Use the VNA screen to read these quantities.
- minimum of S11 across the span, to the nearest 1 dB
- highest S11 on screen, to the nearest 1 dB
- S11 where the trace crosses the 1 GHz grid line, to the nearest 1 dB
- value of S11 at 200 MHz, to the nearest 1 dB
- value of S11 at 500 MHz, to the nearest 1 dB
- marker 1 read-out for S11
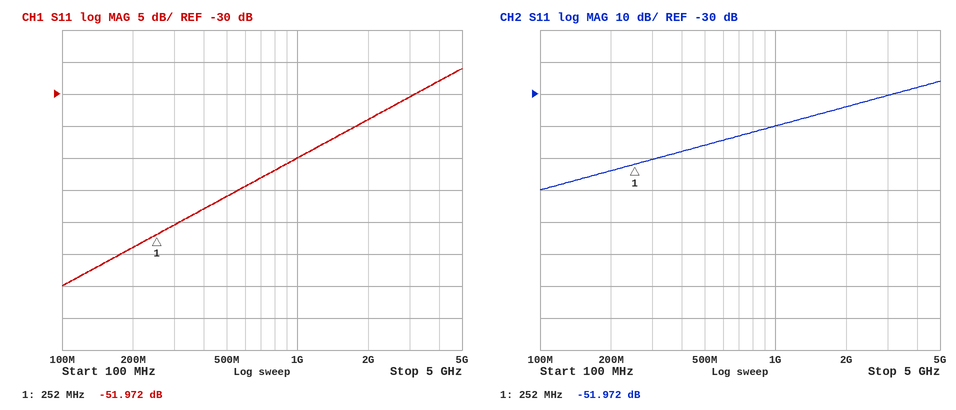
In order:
-60 dB
-26 dB
-40 dB
-54 dB
-46 dB
-51.972 dB
